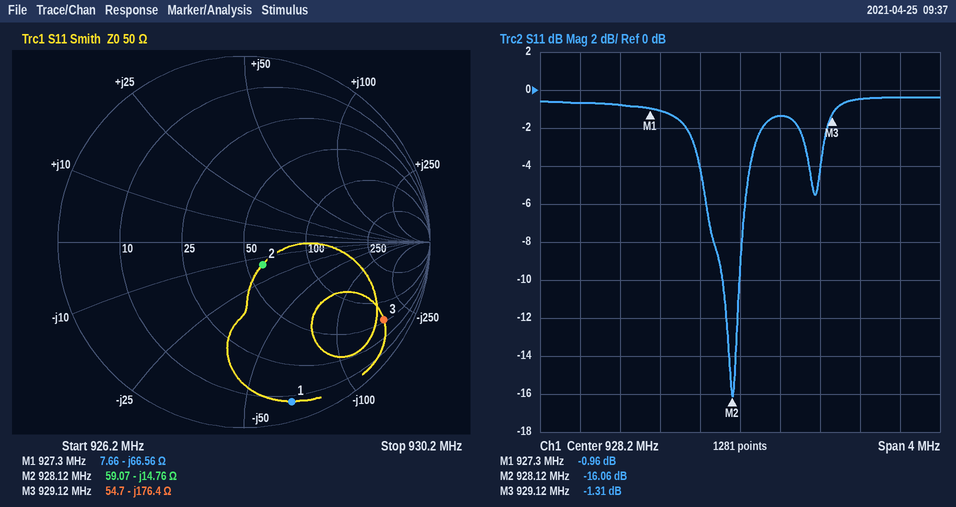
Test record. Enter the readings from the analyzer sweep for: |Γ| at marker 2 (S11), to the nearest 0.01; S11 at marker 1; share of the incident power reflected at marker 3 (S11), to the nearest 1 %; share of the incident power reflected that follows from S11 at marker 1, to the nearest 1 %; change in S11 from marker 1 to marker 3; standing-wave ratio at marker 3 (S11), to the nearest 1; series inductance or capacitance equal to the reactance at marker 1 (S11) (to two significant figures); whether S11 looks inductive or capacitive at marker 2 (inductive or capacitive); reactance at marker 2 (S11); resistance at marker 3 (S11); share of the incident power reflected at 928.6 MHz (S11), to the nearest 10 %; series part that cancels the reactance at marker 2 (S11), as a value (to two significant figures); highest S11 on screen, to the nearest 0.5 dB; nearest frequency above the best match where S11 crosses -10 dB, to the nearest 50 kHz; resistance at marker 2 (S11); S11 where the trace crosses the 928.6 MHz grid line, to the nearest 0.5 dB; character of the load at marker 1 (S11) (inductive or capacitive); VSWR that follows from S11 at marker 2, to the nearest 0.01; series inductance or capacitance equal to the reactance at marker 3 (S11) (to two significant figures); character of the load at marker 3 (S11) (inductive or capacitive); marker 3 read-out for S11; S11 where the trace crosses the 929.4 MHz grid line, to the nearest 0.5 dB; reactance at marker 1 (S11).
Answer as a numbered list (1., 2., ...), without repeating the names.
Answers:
1. 0.16
2. -0.96 dB
3. 74 %
4. 80 %
5. -0.35 dB
6. 13
7. 2.6 pF
8. capacitive
9. -14.76 Ω
10. 54.7 Ω
11. 70 %
12. 2.5 nH
13. -0.5 dB
14. 928.20 MHz
15. 59.07 Ω
16. -1.5 dB
17. capacitive
18. 1.37
19. 970 fF
20. capacitive
21. -1.31 dB
22. -0.5 dB
23. -66.56 Ω
